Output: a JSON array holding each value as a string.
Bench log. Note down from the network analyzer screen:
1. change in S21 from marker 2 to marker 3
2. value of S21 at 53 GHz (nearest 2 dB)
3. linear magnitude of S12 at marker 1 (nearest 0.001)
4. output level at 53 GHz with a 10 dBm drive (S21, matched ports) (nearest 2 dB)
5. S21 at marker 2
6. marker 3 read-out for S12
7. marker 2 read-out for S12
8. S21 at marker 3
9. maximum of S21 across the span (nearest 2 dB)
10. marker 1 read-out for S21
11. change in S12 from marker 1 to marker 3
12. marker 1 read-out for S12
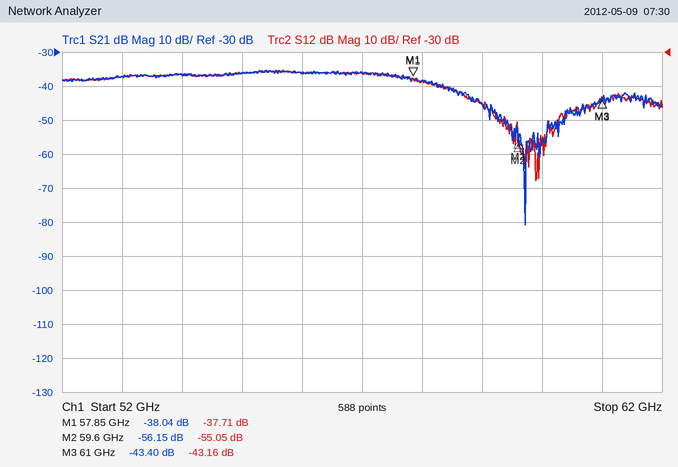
["12.75 dB", "-38 dB", "0.013", "-28 dBm", "-56.15 dB", "-43.16 dB", "-55.05 dB", "-43.40 dB", "-36 dB", "-38.04 dB", "-5.45 dB", "-37.71 dB"]
